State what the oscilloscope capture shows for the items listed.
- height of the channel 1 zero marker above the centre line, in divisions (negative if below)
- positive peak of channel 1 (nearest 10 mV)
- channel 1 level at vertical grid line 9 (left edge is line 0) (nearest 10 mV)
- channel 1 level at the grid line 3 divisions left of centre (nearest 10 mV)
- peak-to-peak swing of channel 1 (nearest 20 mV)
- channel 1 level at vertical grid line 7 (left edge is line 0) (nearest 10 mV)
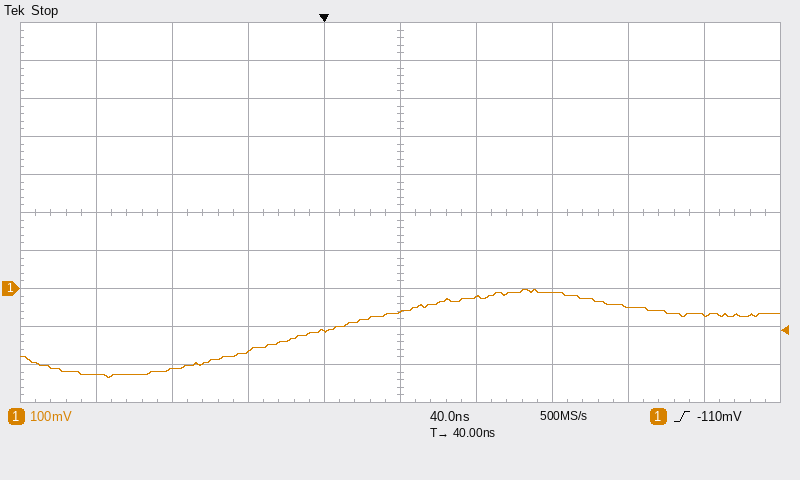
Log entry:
-2.0 div
0 mV
-70 mV
-210 mV
240 mV
-10 mV
